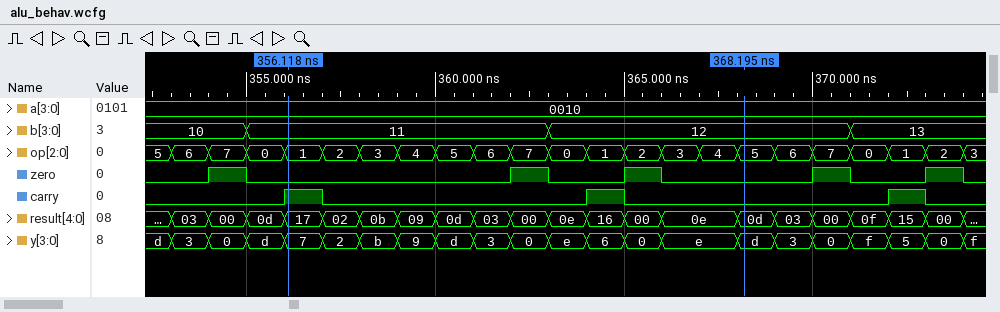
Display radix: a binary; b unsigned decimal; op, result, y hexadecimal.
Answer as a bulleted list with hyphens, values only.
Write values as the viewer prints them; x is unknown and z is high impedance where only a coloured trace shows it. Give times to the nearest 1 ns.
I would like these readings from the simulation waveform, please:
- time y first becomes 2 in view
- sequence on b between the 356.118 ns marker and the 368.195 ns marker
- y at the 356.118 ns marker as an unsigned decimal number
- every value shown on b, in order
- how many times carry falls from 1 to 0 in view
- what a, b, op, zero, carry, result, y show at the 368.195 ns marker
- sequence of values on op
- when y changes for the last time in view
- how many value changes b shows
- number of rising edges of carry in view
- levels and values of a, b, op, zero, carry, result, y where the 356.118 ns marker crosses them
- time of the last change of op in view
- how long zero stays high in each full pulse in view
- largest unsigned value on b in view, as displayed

- 357 ns
- 11, 12
- 7
- 10, 11, 12, 13
- 3
- a=0010, b=12, op=5, zero=0, carry=0, result=0d, y=d
- 5, 6, 7, 0, 1, 2, 3, 4, 5, 6, 7, 0, 1, 2, 3, 4, 5, 6, 7, 0, 1, 2, 3
- 374 ns
- 3
- 3
- a=0010, b=11, op=1, zero=0, carry=1, result=17, y=7
- 374 ns
- 1 ns, 1 ns, 1 ns, 1 ns, 1 ns
- 13
